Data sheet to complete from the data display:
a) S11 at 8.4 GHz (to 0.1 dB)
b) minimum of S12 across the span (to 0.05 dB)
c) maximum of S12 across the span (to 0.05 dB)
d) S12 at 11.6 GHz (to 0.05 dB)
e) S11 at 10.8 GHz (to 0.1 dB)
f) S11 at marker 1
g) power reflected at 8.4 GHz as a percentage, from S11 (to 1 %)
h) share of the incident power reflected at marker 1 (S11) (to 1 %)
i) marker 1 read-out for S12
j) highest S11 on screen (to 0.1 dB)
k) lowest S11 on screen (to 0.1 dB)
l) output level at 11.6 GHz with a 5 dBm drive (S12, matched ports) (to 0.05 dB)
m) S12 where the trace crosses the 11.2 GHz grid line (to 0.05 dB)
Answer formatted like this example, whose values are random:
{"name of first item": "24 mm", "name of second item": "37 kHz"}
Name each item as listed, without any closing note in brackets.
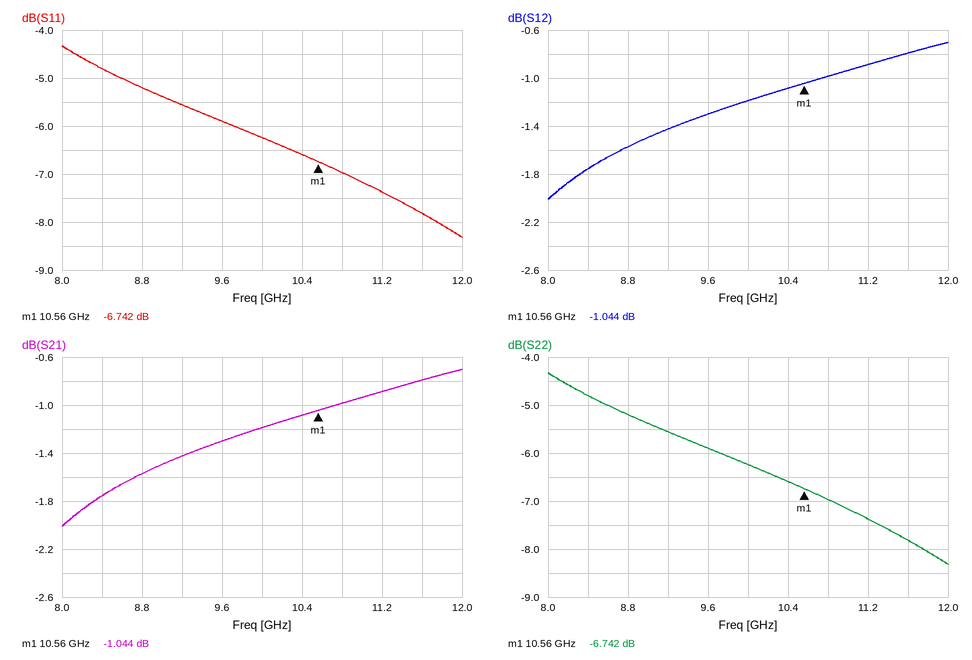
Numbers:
{"S11 at 8.4 GHz": "-4.8 dB", "minimum of S12 across the span": "-2.00 dB", "maximum of S12 across the span": "-0.70 dB", "S12 at 11.6 GHz": "-0.80 dB", "S11 at 10.8 GHz": "-7.0 dB", "S11 at marker 1": "-6.742 dB", "power reflected at 8.4 GHz as a percentage, from S11": "33 %", "share of the incident power reflected at marker 1 (S11)": "21 %", "marker 1 read-out for S12": "-1.044 dB", "highest S11 on screen": "-4.3 dB", "lowest S11 on screen": "-8.3 dB", "output level at 11.6 GHz with a 5 dBm drive (S12, matched ports)": "4.20 dBm", "S12 where the trace crosses the 11.2 GHz grid line": "-0.90 dB"}
